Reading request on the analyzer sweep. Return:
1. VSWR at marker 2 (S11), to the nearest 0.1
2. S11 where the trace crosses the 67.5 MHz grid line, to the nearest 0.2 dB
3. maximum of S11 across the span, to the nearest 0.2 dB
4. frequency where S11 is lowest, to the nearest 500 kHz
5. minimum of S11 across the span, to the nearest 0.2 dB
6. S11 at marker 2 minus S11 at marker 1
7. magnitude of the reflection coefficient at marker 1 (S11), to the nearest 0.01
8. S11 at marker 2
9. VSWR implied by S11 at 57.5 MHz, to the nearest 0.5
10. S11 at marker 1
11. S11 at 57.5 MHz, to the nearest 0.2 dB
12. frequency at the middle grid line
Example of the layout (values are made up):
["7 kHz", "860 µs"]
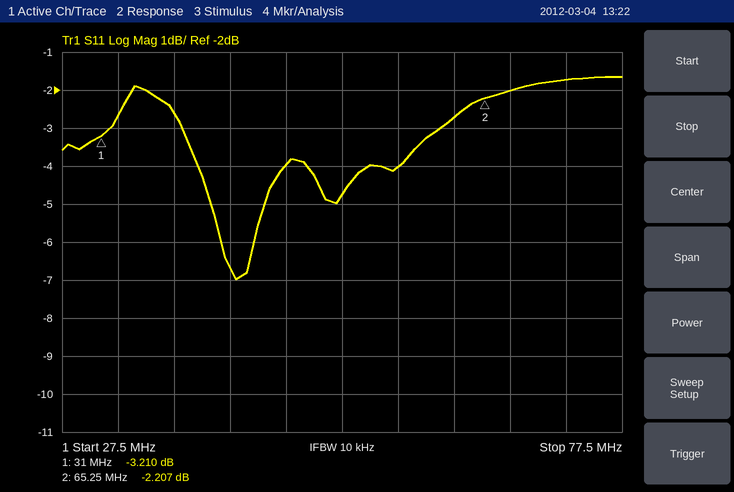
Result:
["7.9", "-2.0 dB", "-1.6 dB", "43.0 MHz", "-7.0 dB", "1.003 dB", "0.69", "-2.207 dB", "4.5", "-3.210 dB", "-4.0 dB", "52.5 MHz"]
